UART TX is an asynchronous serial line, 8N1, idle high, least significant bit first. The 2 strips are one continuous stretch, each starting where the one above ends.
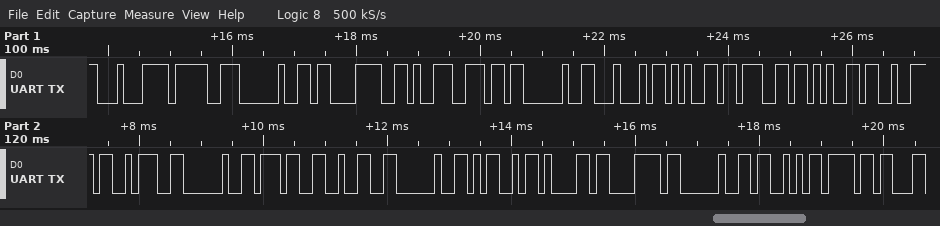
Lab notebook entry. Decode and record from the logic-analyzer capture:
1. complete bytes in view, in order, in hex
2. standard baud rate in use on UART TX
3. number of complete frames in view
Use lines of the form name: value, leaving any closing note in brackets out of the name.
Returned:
complete bytes in view, in order, in hex: 0xC4 0x9F 0x20 0xC3 0x96 0x6E 0x20 0x44 0x65 0x67 0x65 0x72 0x3A 0x20 0x37 0x32 0x20 0x4D 0x61 0x78 0x20 0x53 0x6F
standard baud rate in use on UART TX: 9600 baud
number of complete frames in view: 23
